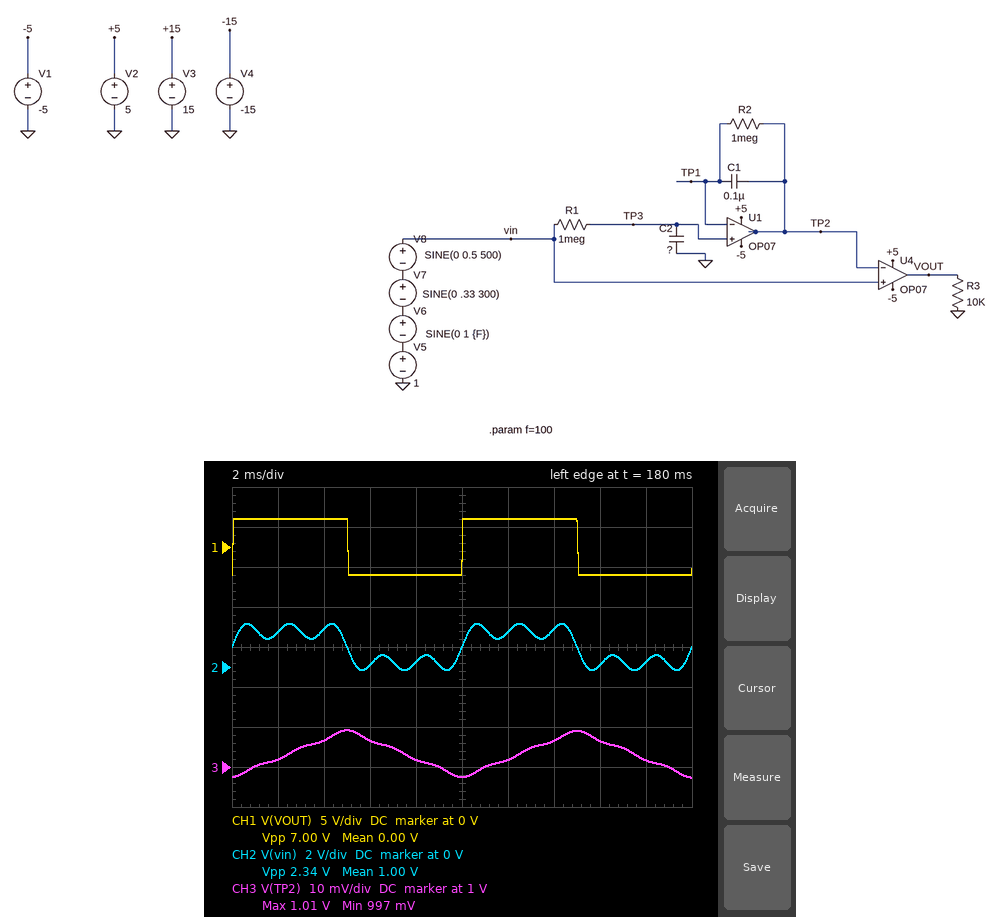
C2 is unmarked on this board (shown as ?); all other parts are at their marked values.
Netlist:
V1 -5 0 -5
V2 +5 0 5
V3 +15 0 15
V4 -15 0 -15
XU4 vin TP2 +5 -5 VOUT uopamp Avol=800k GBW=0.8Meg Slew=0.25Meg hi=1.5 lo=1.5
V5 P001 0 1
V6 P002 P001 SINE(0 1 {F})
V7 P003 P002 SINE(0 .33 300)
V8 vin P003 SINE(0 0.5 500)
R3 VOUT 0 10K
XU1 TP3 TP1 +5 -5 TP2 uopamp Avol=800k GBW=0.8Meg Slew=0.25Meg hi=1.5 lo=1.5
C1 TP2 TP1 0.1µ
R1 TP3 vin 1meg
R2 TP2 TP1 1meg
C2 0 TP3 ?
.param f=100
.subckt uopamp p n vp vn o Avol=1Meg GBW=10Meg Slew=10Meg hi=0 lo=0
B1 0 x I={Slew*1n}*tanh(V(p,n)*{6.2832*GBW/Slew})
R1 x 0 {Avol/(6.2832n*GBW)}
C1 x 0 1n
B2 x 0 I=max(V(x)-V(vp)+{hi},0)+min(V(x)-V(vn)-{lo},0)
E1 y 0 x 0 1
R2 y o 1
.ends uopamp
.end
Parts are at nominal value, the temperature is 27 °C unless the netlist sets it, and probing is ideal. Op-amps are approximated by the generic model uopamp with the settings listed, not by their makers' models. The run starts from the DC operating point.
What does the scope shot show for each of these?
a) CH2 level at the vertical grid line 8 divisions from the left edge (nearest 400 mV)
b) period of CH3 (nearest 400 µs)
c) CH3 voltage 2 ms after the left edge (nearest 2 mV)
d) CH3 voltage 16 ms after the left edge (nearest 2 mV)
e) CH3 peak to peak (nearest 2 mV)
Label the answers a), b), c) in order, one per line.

a) 0 V
b) 10.0 ms
c) 1.002 V
d) 1.006 V
e) 12 mV
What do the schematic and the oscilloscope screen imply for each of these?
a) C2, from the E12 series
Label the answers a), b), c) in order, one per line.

a) 330 nF
